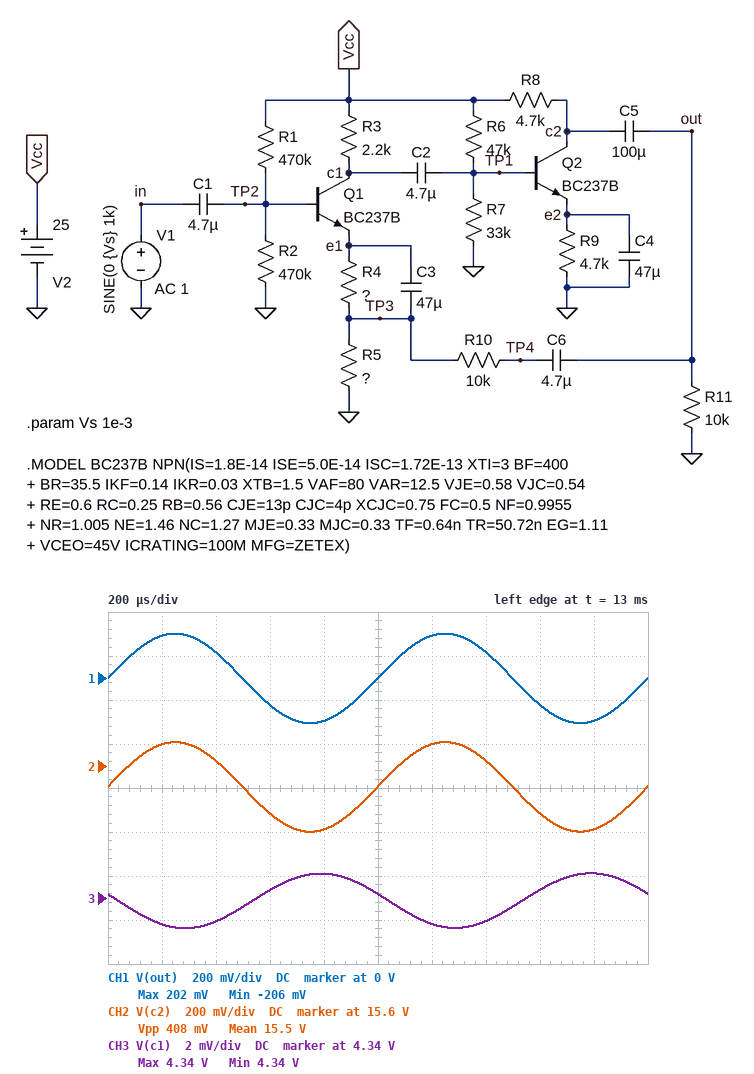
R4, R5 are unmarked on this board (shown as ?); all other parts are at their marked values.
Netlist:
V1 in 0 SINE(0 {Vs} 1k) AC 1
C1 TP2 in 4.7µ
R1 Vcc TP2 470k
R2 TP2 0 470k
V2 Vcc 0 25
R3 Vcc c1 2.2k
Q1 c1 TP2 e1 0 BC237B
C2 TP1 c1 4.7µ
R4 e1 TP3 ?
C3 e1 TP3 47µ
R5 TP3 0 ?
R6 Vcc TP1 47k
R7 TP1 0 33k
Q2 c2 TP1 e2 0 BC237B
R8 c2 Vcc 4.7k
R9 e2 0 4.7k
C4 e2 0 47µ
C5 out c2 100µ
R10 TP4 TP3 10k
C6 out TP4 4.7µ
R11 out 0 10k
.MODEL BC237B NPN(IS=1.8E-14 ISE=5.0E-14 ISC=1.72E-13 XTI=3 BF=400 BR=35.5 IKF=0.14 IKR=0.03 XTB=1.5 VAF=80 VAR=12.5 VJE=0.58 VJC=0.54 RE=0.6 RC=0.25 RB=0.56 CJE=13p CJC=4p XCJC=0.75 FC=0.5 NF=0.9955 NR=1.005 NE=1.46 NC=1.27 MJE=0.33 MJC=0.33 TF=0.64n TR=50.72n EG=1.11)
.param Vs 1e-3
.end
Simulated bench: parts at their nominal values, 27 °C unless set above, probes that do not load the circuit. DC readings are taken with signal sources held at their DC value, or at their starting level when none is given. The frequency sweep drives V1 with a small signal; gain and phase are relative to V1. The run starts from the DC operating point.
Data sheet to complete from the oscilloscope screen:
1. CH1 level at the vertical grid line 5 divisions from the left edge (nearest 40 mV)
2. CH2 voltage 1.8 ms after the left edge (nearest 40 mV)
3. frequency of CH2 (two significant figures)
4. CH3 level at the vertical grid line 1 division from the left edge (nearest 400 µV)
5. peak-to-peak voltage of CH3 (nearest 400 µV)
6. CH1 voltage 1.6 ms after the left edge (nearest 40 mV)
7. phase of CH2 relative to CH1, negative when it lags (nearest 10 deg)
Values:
0 V
15.32 V
1.0 kHz
4.3388 V
2.4 mV
-120 mV
0 deg
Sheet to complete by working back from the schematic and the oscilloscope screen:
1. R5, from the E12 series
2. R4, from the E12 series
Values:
47 Ω
390 Ω
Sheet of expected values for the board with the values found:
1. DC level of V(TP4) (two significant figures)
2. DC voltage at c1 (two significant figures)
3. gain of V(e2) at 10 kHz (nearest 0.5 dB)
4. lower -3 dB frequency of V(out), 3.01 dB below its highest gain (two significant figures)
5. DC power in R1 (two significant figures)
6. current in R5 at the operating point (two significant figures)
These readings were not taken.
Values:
440 mV
4.3 V
-31.0 dB
23 Hz
870 µW
9.4 mA
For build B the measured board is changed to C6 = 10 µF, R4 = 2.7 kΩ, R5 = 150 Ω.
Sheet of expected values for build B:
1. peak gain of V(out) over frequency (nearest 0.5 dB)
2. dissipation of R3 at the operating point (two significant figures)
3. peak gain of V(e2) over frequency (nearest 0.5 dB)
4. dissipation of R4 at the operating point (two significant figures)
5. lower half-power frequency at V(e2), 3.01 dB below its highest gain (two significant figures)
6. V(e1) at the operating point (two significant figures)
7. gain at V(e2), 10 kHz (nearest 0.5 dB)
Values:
41.5 dB
24 mW
21.5 dB
29 mW
10 Hz
9.4 V
-41.0 dB
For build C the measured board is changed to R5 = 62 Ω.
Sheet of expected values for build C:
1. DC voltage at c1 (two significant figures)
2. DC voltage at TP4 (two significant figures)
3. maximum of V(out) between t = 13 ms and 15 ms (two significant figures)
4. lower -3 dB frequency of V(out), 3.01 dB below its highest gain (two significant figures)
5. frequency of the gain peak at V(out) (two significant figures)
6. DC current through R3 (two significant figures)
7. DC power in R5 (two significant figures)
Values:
4.5 V
580 mV
150 mV
19 Hz
25 Hz
9.3 mA
5.4 mW
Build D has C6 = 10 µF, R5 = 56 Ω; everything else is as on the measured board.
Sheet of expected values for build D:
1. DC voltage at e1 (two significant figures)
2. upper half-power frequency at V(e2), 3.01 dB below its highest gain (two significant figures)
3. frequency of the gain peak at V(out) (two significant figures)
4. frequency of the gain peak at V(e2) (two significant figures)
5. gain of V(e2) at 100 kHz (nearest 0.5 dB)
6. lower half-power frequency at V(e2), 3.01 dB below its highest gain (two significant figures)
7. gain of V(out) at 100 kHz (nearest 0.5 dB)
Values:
4.2 V
33 Hz
27 Hz
24 Hz
-52.5 dB
17 Hz
44.5 dB
